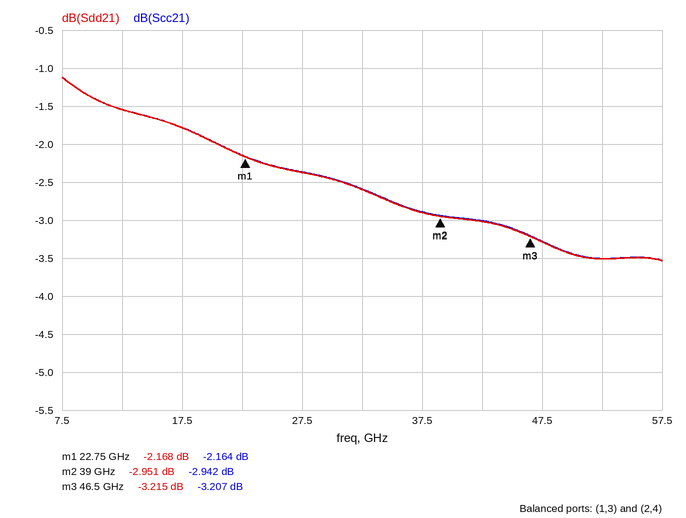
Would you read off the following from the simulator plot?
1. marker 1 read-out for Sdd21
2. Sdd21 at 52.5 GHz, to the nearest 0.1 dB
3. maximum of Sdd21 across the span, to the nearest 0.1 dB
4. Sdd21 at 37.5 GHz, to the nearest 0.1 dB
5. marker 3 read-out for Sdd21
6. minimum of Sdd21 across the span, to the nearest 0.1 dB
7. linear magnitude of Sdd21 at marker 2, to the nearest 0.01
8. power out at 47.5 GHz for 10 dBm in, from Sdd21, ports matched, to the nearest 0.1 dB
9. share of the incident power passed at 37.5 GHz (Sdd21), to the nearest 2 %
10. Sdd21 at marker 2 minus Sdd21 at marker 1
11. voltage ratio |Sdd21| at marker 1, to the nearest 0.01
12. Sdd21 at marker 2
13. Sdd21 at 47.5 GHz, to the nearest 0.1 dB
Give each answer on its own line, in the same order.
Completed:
-2.168 dB
-3.5 dB
-1.1 dB
-2.9 dB
-3.215 dB
-3.5 dB
0.71
6.7 dBm
52 %
-0.783 dB
0.78
-2.951 dB
-3.3 dB
